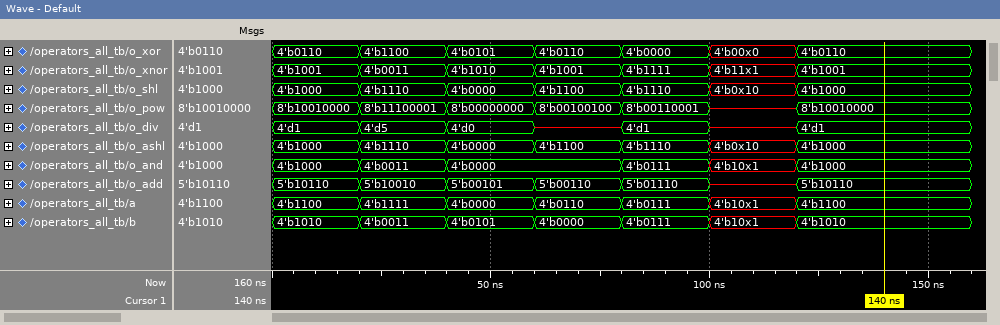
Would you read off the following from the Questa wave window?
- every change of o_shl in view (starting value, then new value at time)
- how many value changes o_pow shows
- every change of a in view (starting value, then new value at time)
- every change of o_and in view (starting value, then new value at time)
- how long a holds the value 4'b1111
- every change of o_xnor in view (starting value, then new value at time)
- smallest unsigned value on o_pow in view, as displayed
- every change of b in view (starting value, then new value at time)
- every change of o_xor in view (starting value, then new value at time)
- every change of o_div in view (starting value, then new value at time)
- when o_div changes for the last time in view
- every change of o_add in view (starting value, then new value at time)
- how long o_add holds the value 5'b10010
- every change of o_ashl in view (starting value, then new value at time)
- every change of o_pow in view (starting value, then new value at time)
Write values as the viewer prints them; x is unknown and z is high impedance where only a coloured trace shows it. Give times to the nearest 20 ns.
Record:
4'b1000, 4'b1110 at 20 ns, 4'b0000 at 40 ns, 4'b1100 at 60 ns, 4'b1110 at 80 ns, 4'b0x10 at 100 ns, 4'b1000 at 120 ns
6
4'b1100, 4'b1111 at 20 ns, 4'b0000 at 40 ns, 4'b0110 at 60 ns, 4'b0111 at 80 ns, 4'b10x1 at 100 ns, 4'b1100 at 120 ns
4'b1000, 4'b0011 at 20 ns, 4'b0000 at 40 ns, 4'b0111 at 80 ns, 4'b10x1 at 100 ns, 4'b1000 at 120 ns
20 ns
4'b1001, 4'b0011 at 20 ns, 4'b1010 at 40 ns, 4'b1001 at 60 ns, 4'b1111 at 80 ns, 4'b11x1 at 100 ns, 4'b1001 at 120 ns
8'b00000000
4'b1010, 4'b0011 at 20 ns, 4'b0101 at 40 ns, 4'b0000 at 60 ns, 4'b0111 at 80 ns, 4'b10x1 at 100 ns, 4'b1010 at 120 ns
4'b0110, 4'b1100 at 20 ns, 4'b0101 at 40 ns, 4'b0110 at 60 ns, 4'b0000 at 80 ns, 4'b00x0 at 100 ns, 4'b0110 at 120 ns
4'd1, 4'd5 at 20 ns, 4'd0 at 40 ns, x at 60 ns, 4'd1 at 80 ns, x at 100 ns, 4'd1 at 120 ns
120 ns
5'b10110, 5'b10010 at 20 ns, 5'b00101 at 40 ns, 5'b00110 at 60 ns, 5'b01110 at 80 ns, x at 100 ns, 5'b10110 at 120 ns
20 ns
4'b1000, 4'b1110 at 20 ns, 4'b0000 at 40 ns, 4'b1100 at 60 ns, 4'b1110 at 80 ns, 4'b0x10 at 100 ns, 4'b1000 at 120 ns
8'b10010000, 8'b11100001 at 20 ns, 8'b00000000 at 40 ns, 8'b00100100 at 60 ns, 8'b00110001 at 80 ns, x at 100 ns, 8'b10010000 at 120 ns
